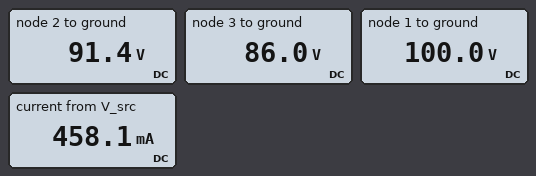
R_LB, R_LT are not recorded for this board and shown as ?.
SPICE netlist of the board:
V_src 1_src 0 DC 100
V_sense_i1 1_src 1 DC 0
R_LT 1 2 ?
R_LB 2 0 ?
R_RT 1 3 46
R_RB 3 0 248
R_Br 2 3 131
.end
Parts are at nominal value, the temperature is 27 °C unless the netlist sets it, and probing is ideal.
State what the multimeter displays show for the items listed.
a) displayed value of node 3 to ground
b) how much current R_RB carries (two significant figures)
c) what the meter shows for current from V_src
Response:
86.0 V
350 mA
458.1 mA
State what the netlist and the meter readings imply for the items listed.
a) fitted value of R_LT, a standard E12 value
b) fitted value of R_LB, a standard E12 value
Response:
56 Ω
820 Ω
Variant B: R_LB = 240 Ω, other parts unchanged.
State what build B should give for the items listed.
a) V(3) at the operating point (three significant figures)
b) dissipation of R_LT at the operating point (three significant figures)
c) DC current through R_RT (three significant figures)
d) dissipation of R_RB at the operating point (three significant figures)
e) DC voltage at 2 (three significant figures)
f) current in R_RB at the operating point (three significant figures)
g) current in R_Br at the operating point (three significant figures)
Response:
83.8 V
5.93 W
353 mA
28.3 W
81.8 V
338 mA
15.2 mA
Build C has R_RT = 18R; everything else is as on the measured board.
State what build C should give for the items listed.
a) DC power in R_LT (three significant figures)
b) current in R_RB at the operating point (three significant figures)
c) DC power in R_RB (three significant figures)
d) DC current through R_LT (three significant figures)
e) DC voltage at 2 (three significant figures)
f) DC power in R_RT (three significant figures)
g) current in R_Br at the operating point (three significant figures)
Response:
752 mW
376 mA
35.1 W
116 mA
93.5 V
2.52 W
1.87 mA
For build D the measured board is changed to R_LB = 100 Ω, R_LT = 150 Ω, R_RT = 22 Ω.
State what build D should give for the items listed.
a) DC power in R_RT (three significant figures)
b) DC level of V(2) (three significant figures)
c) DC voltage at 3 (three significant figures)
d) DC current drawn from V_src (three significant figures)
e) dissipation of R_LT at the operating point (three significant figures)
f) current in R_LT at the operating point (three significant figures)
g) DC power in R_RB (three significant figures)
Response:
7.81 W
54.7 V
86.9 V
898 mA
13.7 W
302 mA
30.4 W
